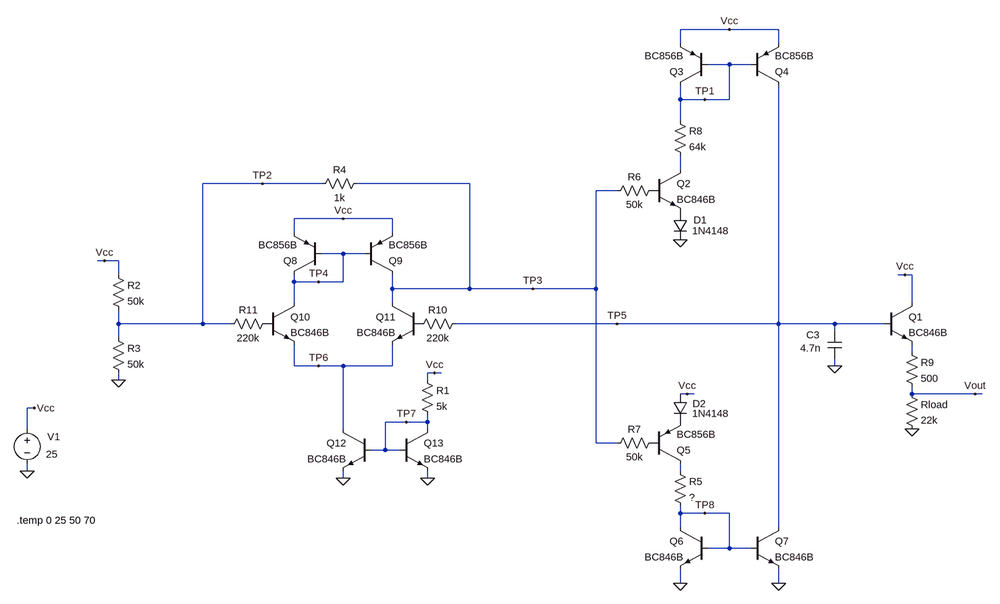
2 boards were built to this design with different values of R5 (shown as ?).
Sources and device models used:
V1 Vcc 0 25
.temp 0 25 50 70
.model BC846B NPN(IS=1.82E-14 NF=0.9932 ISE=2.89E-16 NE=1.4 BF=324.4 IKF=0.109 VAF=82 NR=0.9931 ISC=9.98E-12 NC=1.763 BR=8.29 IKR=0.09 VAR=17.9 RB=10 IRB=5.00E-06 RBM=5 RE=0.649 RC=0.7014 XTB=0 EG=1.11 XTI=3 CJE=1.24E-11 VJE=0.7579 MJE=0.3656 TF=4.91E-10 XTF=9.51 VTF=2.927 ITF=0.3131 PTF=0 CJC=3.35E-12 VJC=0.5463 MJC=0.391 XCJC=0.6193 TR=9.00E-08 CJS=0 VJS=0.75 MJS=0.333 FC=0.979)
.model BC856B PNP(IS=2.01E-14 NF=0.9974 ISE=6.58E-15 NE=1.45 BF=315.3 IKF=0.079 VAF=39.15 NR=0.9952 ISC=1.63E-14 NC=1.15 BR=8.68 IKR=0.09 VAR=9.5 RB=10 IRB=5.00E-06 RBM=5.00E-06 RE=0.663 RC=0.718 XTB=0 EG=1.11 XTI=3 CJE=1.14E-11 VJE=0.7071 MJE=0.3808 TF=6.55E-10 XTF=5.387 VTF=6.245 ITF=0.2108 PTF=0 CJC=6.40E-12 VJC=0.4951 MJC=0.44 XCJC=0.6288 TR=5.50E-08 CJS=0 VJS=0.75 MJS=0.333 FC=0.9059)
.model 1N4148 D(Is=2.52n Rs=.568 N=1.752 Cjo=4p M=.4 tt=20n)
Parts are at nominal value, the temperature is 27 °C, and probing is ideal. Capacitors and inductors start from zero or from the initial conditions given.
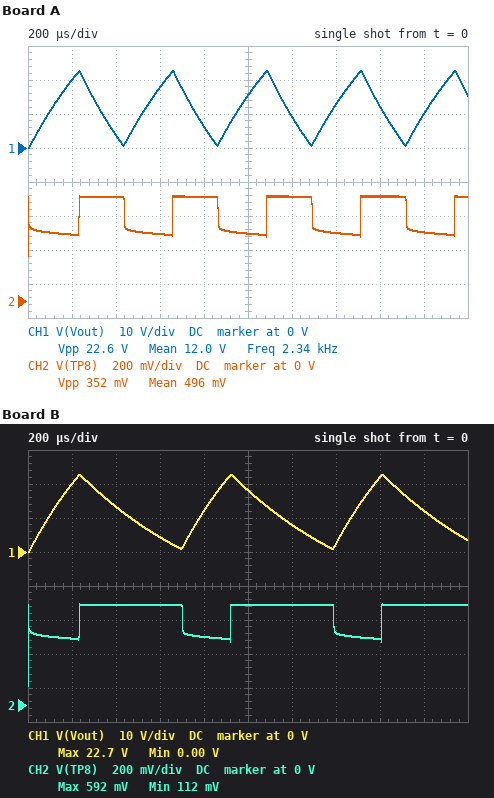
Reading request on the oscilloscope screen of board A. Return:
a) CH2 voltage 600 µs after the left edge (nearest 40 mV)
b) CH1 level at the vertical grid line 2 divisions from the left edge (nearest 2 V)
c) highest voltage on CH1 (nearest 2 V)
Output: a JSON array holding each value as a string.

["400 mV", "4 V", "22 V"]
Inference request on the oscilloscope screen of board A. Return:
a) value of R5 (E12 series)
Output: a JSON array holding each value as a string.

["56 kΩ"]
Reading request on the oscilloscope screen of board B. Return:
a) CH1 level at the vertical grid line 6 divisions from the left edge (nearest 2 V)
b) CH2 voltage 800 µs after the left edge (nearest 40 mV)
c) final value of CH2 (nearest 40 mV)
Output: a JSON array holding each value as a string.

["8 V", "400 mV", "600 mV"]
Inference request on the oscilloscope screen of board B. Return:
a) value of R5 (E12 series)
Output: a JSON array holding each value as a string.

["150 kΩ"]
